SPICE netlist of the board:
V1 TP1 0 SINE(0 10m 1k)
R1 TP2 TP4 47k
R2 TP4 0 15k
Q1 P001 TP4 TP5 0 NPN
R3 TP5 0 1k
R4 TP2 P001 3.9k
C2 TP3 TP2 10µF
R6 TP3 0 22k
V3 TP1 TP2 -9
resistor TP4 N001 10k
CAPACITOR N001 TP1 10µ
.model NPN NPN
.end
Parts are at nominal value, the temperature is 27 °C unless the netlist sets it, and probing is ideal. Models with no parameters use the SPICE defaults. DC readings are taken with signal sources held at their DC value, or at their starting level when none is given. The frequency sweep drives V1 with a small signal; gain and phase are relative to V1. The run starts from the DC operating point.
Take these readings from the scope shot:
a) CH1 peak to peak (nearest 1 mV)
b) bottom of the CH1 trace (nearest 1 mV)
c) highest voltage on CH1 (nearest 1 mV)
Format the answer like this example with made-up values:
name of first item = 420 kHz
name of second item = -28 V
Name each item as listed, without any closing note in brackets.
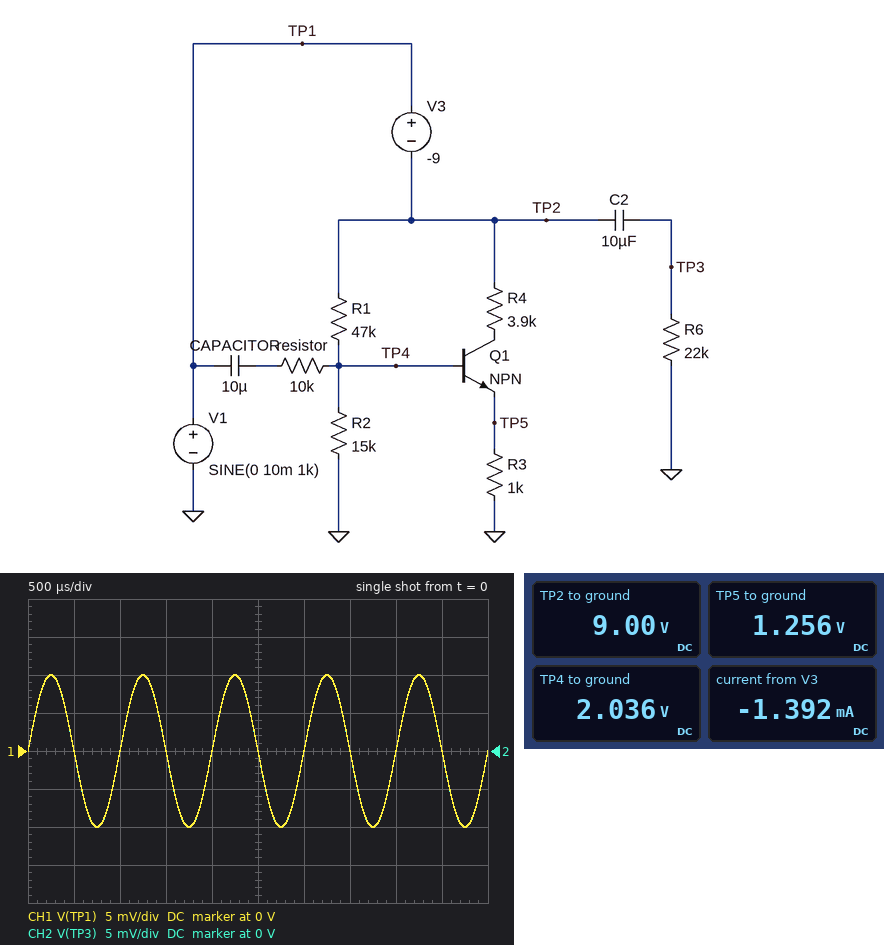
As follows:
CH1 peak to peak = 20 mV
bottom of the CH1 trace = -10 mV
highest voltage on CH1 = 10 mV
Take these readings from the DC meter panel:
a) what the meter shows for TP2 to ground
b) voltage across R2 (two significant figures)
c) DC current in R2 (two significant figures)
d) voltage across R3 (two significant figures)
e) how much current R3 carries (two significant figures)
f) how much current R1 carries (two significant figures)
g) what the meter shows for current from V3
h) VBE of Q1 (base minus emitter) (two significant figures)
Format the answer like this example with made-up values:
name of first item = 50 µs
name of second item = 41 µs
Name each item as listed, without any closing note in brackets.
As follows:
what the meter shows for TP2 to ground = 9.00 V
voltage across R2 = 2.0 V
DC current in R2 = 140 µA
voltage across R3 = 1.3 V
how much current R3 carries = 1.3 mA
how much current R1 carries = 150 µA
what the meter shows for current from V3 = -1.392 mA
VBE of Q1 (base minus emitter) = 780 mV
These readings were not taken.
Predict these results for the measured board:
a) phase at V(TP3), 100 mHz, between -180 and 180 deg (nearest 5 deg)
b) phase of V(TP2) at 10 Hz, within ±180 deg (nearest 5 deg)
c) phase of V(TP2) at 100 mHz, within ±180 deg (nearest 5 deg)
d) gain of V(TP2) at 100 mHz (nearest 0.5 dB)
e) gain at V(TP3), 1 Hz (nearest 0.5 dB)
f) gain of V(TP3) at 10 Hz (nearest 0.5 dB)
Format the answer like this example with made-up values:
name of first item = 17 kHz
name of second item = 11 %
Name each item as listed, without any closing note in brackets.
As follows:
phase at V(TP3), 100 mHz, between -180 and 180 deg = 80 deg
phase of V(TP2) at 10 Hz, within ±180 deg = 0 deg
phase of V(TP2) at 100 mHz, within ±180 deg = 0 deg
gain of V(TP2) at 100 mHz = 0 dB
gain at V(TP3), 1 Hz = -2.0 dB
gain of V(TP3) at 10 Hz = 0 dB
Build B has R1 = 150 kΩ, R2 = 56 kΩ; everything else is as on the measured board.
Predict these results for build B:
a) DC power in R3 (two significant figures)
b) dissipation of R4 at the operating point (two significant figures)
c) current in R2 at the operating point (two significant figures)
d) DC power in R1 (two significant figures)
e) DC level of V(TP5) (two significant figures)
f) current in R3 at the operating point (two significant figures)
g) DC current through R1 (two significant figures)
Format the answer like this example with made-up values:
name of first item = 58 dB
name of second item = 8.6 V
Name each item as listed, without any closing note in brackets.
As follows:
DC power in R3 = 1.4 mW
dissipation of R4 at the operating point = 5.4 mW
current in R2 at the operating point = 35 µA
DC power in R1 = 330 µW
DC level of V(TP5) = 1.2 V
current in R3 at the operating point = 1.2 mA
DC current through R1 = 47 µA
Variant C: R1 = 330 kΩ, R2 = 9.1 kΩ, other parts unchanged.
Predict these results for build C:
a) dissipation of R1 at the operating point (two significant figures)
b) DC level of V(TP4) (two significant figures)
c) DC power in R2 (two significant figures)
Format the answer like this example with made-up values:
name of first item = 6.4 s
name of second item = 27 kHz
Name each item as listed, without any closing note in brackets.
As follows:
dissipation of R1 at the operating point = 230 µW
DC level of V(TP4) = 240 mV
DC power in R2 = 6.4 µW
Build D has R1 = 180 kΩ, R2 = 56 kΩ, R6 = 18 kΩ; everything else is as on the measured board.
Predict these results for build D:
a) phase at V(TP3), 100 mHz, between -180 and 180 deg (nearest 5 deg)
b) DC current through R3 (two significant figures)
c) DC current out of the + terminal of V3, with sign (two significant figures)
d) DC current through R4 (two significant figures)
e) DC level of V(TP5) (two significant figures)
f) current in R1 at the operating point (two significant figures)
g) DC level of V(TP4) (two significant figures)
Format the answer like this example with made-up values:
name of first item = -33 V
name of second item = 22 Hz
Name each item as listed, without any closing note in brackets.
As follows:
phase at V(TP3), 100 mHz, between -180 and 180 deg = 85 deg
DC current through R3 = 960 µA
DC current out of the + terminal of V3, with sign = -990 µA
DC current through R4 = 950 µA
DC level of V(TP5) = 960 mV
current in R1 at the operating point = 40 µA
DC level of V(TP4) = 1.7 V
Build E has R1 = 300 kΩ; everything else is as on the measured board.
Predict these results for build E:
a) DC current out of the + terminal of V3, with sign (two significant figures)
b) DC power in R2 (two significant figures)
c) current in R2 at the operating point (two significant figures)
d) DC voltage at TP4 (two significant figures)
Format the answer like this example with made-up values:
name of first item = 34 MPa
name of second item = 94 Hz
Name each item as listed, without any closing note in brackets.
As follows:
DC current out of the + terminal of V3, with sign = -29 µA
DC power in R2 = 12 µW
current in R2 at the operating point = 29 µA
DC voltage at TP4 = 430 mV
